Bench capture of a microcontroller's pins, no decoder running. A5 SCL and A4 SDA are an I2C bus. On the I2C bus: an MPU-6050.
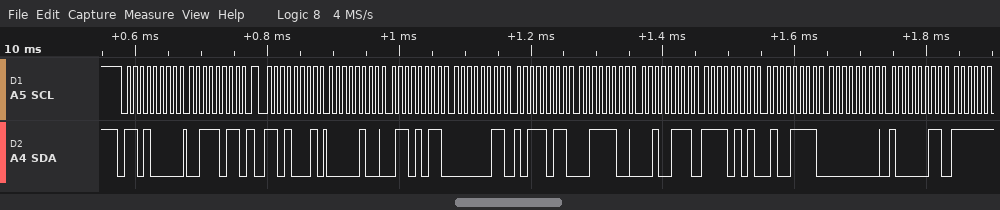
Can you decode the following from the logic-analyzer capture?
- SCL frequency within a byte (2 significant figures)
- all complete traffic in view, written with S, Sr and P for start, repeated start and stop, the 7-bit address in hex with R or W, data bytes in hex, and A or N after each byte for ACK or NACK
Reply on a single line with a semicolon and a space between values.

100 kHz; S 68W A 3B A Sr 68R A 04 A 6B A 03 A BB A 3C A 27 A F5 A 4F A 00 A 83 A
